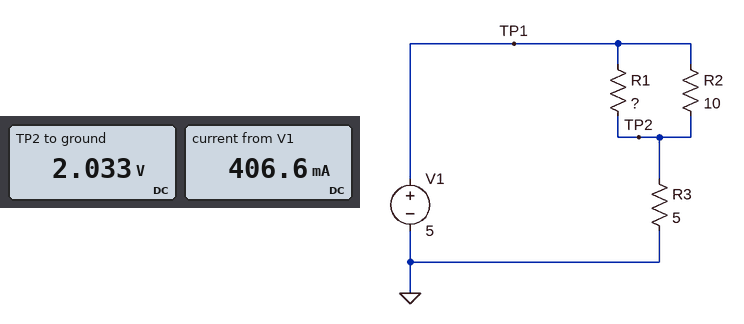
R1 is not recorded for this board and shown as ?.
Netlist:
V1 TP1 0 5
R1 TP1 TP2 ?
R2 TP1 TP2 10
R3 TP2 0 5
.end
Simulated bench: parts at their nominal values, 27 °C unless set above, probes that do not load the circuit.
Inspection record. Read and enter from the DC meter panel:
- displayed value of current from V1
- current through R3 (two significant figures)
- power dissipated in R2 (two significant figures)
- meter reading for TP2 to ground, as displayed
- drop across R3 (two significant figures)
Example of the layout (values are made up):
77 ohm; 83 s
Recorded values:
406.6 mA; 410 mA; 880 mW; 2.033 V; 2.0 V
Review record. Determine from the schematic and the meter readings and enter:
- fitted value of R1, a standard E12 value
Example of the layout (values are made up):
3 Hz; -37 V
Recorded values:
27 Ω
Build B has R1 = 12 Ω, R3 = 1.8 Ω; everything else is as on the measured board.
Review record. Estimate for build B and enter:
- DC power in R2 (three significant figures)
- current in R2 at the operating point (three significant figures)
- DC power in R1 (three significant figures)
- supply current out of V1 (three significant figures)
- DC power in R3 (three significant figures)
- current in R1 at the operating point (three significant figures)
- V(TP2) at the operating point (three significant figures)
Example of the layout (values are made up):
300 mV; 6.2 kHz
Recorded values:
1.41 W; 376 mA; 1.18 W; 689 mA; 855 mW; 313 mA; 1.24 V
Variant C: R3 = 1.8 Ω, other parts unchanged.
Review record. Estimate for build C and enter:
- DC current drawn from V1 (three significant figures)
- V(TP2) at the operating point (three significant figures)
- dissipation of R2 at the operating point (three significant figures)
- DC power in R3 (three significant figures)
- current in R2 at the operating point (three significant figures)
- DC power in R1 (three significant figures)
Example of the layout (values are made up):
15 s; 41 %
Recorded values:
550 mA; 989 mV; 1.61 W; 544 mW; 401 mA; 596 mW
